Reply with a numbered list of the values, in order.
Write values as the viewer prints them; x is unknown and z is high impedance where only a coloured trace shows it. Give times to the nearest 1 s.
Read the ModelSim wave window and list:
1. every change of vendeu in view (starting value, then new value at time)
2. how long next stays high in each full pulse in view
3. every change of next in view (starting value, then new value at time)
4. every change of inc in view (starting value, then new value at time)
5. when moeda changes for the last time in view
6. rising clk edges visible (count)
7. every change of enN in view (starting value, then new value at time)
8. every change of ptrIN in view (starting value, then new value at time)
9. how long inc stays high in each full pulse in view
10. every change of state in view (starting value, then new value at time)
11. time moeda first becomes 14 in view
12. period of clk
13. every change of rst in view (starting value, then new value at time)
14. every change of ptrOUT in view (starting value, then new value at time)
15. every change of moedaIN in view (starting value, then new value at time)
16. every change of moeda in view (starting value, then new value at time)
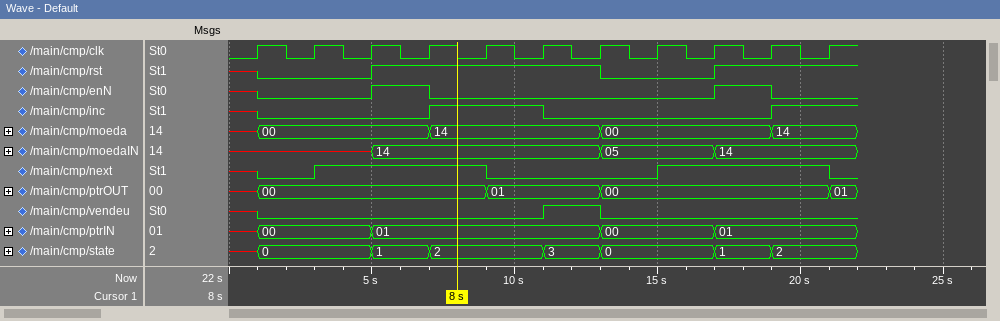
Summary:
1. x, 0 at 1 s, 1 at 11 s, 0 at 13 s
2. 6 s, 6 s
3. x, 0 at 1 s, 1 at 3 s, 0 at 9 s, 1 at 15 s, 0 at 21 s
4. x, 0 at 1 s, 1 at 7 s, 0 at 11 s, 1 at 19 s
5. 19 s
6. 11
7. x, 0 at 1 s, 1 at 5 s, 0 at 7 s, 1 at 17 s, 0 at 19 s
8. x, 00 at 1 s, 01 at 5 s, 00 at 13 s, 01 at 17 s
9. 4 s
10. x, 0 at 1 s, 1 at 5 s, 2 at 7 s, 3 at 11 s, 0 at 13 s, 1 at 17 s, 2 at 19 s
11. 7 s
12. 2 s
13. x, 0 at 1 s, 1 at 5 s, 0 at 13 s, 1 at 17 s
14. x, 00 at 1 s, 01 at 9 s, 00 at 13 s, 01 at 21 s
15. x, 14 at 5 s, 05 at 13 s, 14 at 17 s
16. x, 00 at 1 s, 14 at 7 s, 00 at 13 s, 14 at 19 s
